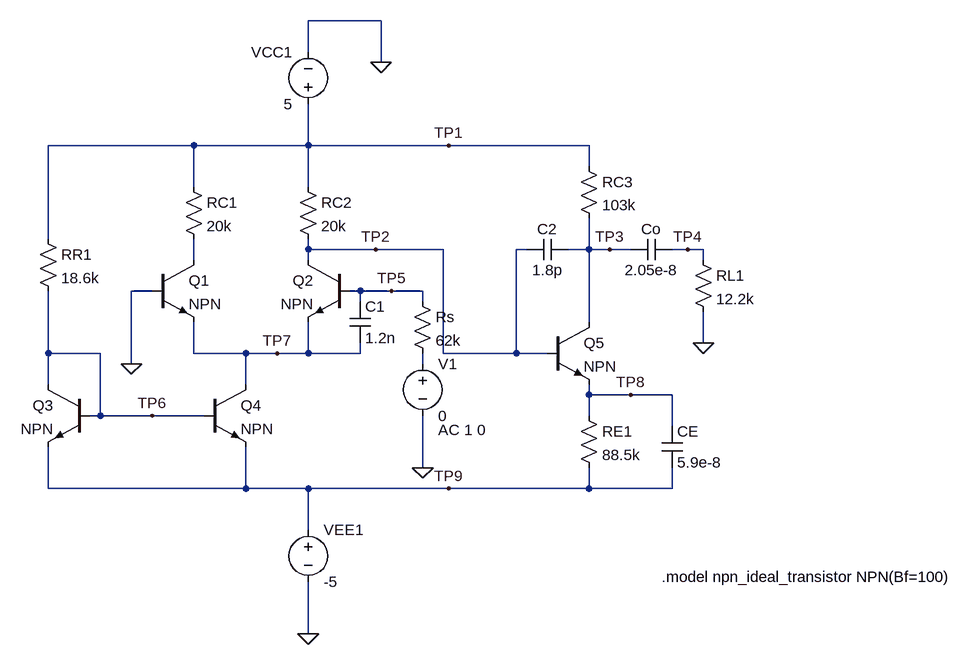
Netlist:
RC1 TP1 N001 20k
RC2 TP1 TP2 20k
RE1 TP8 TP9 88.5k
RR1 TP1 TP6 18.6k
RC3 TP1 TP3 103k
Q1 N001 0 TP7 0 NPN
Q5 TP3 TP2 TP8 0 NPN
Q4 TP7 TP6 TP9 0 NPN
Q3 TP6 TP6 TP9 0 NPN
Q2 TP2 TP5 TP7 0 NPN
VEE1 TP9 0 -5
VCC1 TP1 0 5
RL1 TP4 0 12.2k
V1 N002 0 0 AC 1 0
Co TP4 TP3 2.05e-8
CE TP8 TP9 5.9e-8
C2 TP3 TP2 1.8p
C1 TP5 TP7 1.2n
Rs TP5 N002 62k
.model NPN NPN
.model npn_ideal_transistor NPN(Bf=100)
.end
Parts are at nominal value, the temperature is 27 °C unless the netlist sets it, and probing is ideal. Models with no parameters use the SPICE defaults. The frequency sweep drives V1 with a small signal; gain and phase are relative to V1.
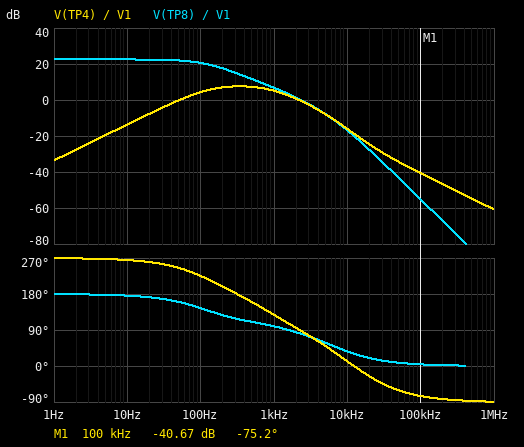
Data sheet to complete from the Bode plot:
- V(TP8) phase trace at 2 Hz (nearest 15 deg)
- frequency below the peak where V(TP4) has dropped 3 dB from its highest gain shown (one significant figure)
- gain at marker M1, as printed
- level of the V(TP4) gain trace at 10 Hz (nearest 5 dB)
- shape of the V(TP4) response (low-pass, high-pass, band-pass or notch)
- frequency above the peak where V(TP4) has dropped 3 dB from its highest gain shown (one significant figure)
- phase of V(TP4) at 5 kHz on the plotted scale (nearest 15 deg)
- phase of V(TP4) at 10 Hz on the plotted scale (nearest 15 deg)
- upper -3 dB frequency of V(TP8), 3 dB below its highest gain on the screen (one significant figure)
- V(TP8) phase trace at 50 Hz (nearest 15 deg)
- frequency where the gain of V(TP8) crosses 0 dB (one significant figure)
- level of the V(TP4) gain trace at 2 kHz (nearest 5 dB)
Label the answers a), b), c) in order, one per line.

a) 180 deg
b) 100 Hz
c) -40.67 dB
d) -15 dB
e) band-pass
f) 1 kHz
g) 45 deg
h) 270 deg
i) 100 Hz
j) 165 deg
k) 2 kHz
l) 0 dB
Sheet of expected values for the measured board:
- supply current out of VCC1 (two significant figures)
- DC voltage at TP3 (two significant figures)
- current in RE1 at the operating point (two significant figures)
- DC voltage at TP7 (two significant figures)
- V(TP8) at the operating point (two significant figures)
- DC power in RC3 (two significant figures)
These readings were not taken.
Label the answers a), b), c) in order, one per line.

a) 940 µA
b) 1.8 V
c) 77 µA
d) -760 mV
e) 1.8 V
f) 98 µW
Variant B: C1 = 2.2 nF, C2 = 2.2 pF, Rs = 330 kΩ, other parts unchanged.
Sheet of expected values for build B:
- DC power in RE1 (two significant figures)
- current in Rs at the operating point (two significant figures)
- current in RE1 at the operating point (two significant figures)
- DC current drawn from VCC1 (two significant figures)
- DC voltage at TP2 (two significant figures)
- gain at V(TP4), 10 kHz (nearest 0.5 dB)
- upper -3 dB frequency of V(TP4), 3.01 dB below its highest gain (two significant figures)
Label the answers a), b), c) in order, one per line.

a) 640 µW
b) 250 nA
c) 85 µA
d) 890 µA
e) 3.3 V
f) -45.0 dB
g) 760 Hz
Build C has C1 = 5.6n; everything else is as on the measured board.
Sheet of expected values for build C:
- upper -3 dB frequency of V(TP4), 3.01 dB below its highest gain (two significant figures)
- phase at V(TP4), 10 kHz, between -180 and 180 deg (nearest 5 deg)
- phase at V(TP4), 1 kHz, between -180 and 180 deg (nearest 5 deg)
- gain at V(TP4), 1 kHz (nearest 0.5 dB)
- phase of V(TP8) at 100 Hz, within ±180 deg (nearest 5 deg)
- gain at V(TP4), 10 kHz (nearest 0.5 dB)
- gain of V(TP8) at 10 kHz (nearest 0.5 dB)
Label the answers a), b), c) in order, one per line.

a) 890 Hz
b) -15 deg
c) 100 deg
d) 3.5 dB
e) 140 deg
f) -28.0 dB
g) -28.5 dB
